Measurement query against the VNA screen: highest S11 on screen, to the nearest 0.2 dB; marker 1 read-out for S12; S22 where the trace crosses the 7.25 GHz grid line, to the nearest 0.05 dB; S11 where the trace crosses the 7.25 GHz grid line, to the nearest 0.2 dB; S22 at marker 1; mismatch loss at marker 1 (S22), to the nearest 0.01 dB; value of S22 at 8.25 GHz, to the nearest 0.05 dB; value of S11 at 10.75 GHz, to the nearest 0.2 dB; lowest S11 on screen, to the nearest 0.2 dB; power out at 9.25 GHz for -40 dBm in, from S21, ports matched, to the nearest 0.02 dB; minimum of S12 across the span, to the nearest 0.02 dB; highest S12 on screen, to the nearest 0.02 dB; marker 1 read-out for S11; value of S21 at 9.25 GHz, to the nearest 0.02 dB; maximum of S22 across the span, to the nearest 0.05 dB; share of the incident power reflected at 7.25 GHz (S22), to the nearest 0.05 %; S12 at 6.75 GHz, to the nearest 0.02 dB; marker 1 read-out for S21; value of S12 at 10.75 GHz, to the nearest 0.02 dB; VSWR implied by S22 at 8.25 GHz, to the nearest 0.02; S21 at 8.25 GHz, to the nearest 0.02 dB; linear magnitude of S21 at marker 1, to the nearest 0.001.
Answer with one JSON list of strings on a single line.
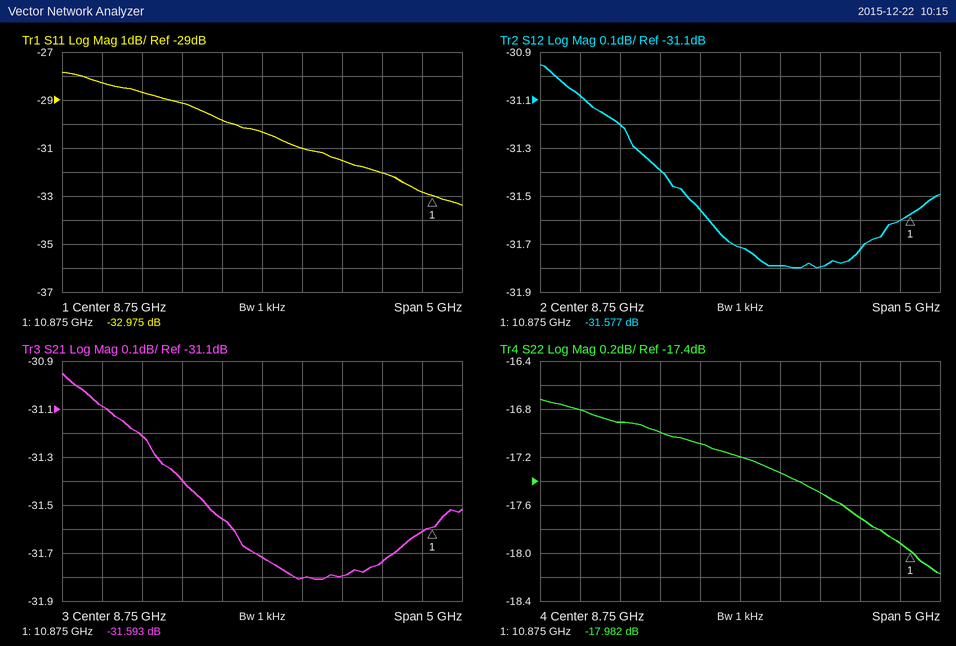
["-27.8 dB", "-31.577 dB", "-16.90 dB", "-28.6 dB", "-17.982 dB", "0.07 dB", "-17.10 dB", "-32.8 dB", "-33.4 dB", "-71.80 dBm", "-31.80 dB", "-30.96 dB", "-32.975 dB", "-31.80 dB", "-16.70 dB", "2.05 %", "-31.08 dB", "-31.593 dB", "-31.60 dB", "1.32", "-31.56 dB", "0.026"]
